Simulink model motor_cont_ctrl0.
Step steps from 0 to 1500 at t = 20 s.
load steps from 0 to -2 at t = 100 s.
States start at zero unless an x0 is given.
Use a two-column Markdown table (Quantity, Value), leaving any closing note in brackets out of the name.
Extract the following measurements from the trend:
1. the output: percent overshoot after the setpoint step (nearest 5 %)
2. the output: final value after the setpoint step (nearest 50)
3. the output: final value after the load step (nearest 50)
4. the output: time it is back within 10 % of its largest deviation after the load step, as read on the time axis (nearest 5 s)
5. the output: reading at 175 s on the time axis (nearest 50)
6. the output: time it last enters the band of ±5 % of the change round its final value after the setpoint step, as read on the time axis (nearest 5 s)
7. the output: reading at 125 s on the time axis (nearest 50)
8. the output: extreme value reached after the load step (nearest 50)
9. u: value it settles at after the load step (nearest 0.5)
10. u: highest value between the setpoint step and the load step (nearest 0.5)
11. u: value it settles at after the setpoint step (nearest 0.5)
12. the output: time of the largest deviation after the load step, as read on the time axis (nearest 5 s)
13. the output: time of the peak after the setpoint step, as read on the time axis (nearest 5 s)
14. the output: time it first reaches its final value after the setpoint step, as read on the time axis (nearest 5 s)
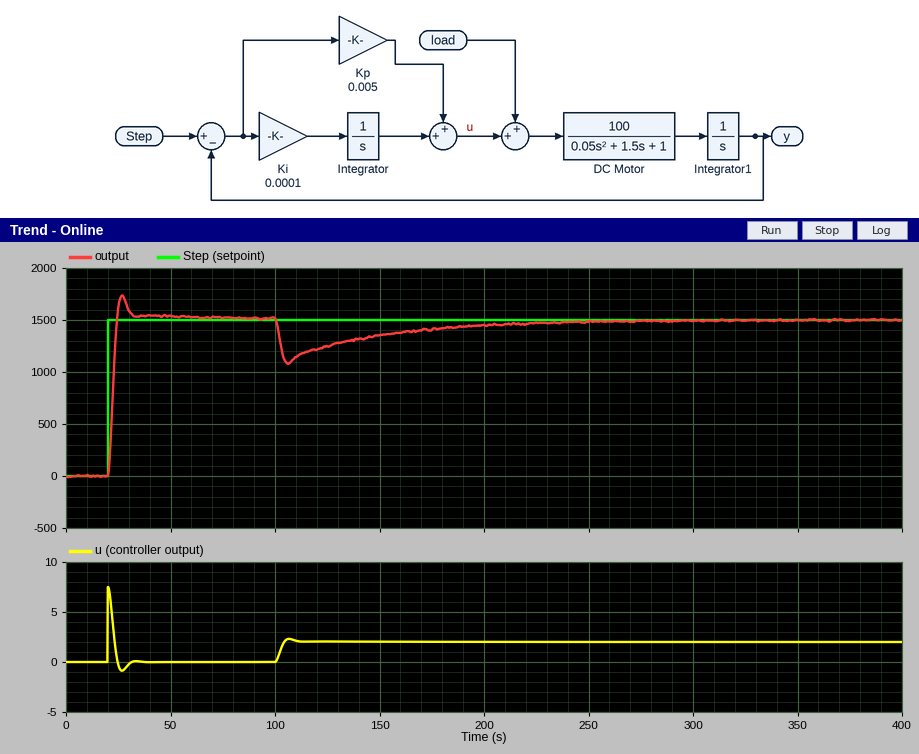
| Quantity | Value |
|---|---|
| the output: percent overshoot after the setpoint step | 15 % |
| the output: final value after the setpoint step | 1500 |
| the output: final value after the load step | 1500 |
| the output: time it is back within 10 % of its largest deviation after the load step, as read on the time axis | 210 s |
| the output: reading at 175 s on the time axis | 1400 |
| the output: time it last enters the band of ±5 % of the change round its final value after the setpoint step, as read on the time axis | 30 s |
| the output: reading at 125 s on the time axis | 1250 |
| the output: extreme value reached after the load step | 1100 |
| u: value it settles at after the load step | 2.0 |
| u: highest value between the setpoint step and the load step | 7.5 |
| u: value it settles at after the setpoint step | 0.0 |
| the output: time of the largest deviation after the load step, as read on the time axis | 105 s |
| the output: time of the peak after the setpoint step, as read on the time axis | 25 s |
| the output: time it first reaches its final value after the setpoint step, as read on the time axis | 25 s |
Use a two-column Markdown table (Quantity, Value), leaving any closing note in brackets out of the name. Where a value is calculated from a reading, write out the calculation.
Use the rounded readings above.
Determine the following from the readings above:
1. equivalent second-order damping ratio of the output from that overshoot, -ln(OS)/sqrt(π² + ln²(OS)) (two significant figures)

| Quantity | Value |
|---|---|
| equivalent second-order damping ratio of the output from that overshoot, -ln(OS)/sqrt(π² + ln²(OS)) | ln(0.15) = -1.897; 1.897 / sqrt(9.870 + 3.599) = 0.52 |
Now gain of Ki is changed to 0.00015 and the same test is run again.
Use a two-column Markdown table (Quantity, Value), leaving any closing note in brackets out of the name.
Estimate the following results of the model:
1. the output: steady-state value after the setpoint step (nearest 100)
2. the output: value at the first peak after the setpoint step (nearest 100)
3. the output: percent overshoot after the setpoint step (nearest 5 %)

| Quantity | Value |
|---|---|
| the output: steady-state value after the setpoint step | 1500 |
| the output: value at the first peak after the setpoint step | 1800 |
| the output: percent overshoot after the setpoint step | 20 % |
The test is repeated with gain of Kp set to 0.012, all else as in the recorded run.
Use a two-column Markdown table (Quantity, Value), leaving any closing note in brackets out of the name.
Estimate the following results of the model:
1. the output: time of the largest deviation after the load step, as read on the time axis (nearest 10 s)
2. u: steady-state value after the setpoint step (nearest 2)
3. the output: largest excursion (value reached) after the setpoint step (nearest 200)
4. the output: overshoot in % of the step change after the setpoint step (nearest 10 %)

| Quantity | Value |
|---|---|
| the output: time of the largest deviation after the load step, as read on the time axis | 100 s |
| u: steady-state value after the setpoint step | 0 |
| the output: largest excursion (value reached) after the setpoint step | 2000 |
| the output: overshoot in % of the step change after the setpoint step | 30 % |
